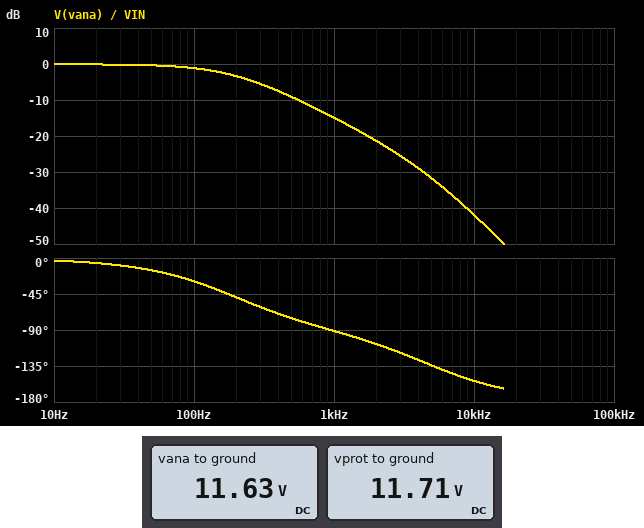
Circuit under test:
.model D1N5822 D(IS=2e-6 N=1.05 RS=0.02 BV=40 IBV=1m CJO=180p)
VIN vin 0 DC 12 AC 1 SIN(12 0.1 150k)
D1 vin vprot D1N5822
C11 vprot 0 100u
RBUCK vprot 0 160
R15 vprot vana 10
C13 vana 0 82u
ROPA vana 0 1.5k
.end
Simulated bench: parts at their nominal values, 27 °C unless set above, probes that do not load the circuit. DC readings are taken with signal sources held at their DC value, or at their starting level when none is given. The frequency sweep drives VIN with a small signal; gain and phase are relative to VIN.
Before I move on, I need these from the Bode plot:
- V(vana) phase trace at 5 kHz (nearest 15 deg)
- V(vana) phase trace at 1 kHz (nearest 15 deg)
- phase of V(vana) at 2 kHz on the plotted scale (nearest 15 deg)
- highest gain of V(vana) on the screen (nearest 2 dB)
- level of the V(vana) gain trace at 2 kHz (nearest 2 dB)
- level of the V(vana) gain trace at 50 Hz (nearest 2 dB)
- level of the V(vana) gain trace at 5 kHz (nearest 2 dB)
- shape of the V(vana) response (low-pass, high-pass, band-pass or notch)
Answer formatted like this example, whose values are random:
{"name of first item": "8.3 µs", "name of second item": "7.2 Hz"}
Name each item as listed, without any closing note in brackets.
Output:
{"V(vana) phase trace at 5 kHz": "-135 deg", "V(vana) phase trace at 1 kHz": "-90 deg", "phase of V(vana) at 2 kHz on the plotted scale": "-105 deg", "highest gain of V(vana) on the screen": "0 dB", "level of the V(vana) gain trace at 2 kHz": "-22 dB", "level of the V(vana) gain trace at 50 Hz": "0 dB", "level of the V(vana) gain trace at 5 kHz": "-32 dB", "shape of the V(vana) response": "low-pass"}
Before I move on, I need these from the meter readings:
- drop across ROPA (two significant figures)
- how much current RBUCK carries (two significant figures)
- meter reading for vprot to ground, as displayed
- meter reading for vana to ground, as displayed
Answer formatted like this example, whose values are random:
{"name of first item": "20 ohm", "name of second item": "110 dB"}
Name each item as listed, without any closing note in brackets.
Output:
{"drop across ROPA": "12 V", "how much current RBUCK carries": "73 mA", "meter reading for vprot to ground, as displayed": "11.71 V", "meter reading for vana to ground, as displayed": "11.63 V"}
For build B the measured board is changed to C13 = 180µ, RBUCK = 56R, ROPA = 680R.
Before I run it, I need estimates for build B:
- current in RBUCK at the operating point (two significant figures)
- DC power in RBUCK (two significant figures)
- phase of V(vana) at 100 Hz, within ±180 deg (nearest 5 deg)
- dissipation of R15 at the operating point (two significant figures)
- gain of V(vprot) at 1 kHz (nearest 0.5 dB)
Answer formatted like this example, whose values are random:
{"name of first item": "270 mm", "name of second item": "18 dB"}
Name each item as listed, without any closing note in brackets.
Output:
{"current in RBUCK at the operating point": "210 mA", "DC power in RBUCK": "2.4 W", "phase of V(vana) at 100 Hz, within ±180 deg": "-50 deg", "dissipation of R15 at the operating point": "2.9 mW", "gain of V(vprot) at 1 kHz": "0 dB"}
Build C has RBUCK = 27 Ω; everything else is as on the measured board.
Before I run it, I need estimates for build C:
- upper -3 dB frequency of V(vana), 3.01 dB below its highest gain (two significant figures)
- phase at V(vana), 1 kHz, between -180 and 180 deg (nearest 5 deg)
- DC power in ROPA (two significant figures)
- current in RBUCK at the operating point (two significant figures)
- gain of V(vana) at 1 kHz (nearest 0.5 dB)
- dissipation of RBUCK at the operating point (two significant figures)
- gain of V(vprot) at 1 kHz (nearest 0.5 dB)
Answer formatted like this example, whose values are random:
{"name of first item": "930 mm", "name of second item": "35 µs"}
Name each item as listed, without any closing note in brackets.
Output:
{"upper -3 dB frequency of V(vana), 3.01 dB below its highest gain": "190 Hz", "phase at V(vana), 1 kHz, between -180 and 180 deg": "-80 deg", "DC power in ROPA": "89 mW", "current in RBUCK at the operating point": "430 mA", "gain of V(vana) at 1 kHz": "-14.5 dB", "dissipation of RBUCK at the operating point": "5.0 W", "gain of V(vprot) at 1 kHz": "0 dB"}
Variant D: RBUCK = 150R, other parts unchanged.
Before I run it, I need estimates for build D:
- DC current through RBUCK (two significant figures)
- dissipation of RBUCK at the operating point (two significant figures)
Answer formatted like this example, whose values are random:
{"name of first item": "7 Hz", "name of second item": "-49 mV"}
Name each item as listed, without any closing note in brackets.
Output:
{"DC current through RBUCK": "78 mA", "dissipation of RBUCK at the operating point": "910 mW"}
